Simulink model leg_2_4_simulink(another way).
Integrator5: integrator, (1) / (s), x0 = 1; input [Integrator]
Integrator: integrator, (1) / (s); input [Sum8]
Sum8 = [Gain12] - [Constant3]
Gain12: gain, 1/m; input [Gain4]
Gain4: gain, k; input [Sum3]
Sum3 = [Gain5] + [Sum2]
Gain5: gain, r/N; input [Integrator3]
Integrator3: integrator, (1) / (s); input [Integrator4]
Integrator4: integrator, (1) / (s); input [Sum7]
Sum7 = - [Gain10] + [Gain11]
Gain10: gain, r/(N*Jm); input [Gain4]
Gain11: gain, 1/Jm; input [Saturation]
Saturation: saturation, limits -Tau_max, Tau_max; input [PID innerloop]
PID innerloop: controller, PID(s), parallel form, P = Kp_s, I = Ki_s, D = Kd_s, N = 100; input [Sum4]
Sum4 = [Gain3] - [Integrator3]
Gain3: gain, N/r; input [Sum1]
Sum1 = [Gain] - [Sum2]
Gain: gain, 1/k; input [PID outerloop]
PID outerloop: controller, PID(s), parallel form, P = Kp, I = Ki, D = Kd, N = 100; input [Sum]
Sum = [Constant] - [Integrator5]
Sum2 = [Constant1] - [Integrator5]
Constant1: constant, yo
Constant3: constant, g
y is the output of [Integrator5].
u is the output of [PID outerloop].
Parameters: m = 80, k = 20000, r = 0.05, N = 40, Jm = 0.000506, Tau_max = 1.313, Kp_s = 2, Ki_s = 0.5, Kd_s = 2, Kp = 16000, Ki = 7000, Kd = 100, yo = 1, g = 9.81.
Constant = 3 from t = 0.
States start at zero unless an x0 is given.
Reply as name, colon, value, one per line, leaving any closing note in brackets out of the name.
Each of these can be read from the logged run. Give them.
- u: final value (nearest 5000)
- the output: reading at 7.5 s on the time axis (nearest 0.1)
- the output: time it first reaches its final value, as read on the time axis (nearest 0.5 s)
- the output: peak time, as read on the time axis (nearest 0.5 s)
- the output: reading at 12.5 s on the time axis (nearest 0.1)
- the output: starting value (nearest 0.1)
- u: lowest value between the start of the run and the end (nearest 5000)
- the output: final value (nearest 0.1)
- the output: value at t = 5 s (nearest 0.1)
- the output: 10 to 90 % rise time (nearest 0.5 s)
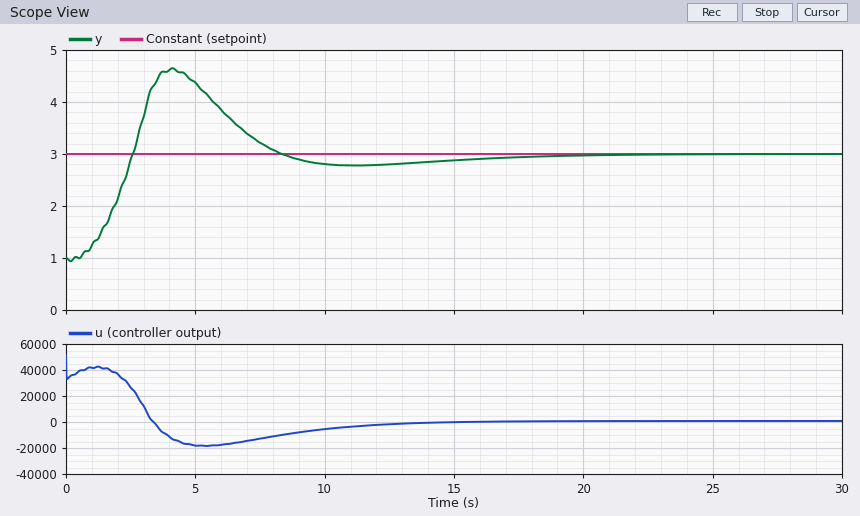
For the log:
u: final value: 0
the output: reading at 7.5 s on the time axis: 3.2
the output: time it first reaches its final value, as read on the time axis: 2.5 s
the output: peak time, as read on the time axis: 4.0 s
the output: reading at 12.5 s on the time axis: 2.8
the output: starting value: 1.0
u: lowest value between the start of the run and the end: -20000
the output: final value: 3.0
the output: value at t = 5 s: 4.4
the output: 10 to 90 % rise time: 1.5 s
